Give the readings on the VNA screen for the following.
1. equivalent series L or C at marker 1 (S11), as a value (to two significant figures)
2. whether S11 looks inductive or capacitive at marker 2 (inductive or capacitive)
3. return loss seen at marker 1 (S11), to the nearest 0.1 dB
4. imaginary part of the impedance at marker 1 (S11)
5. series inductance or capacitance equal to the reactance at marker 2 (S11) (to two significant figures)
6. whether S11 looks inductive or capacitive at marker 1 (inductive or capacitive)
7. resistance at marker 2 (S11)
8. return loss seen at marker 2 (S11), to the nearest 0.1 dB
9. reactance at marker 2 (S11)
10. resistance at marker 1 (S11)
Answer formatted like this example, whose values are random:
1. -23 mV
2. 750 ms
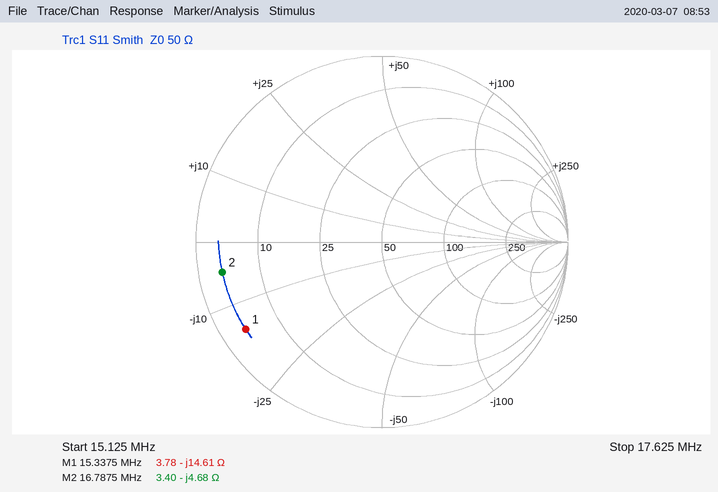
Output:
1. 710 pF
2. capacitive
3. 1.2 dB
4. -14.61 Ω
5. 2.0 nF
6. capacitive
7. 3.40 Ω
8. 1.2 dB
9. -4.68 Ω
10. 3.78 Ω
